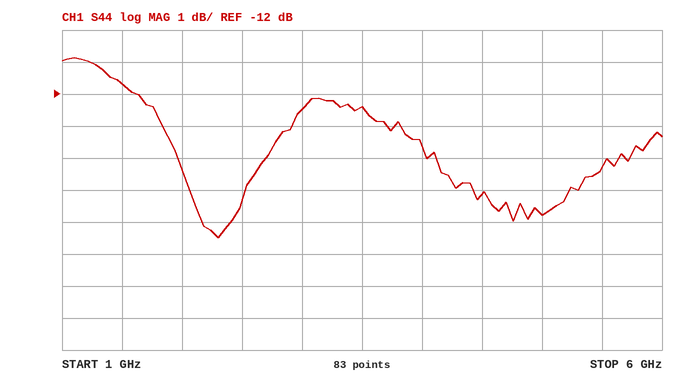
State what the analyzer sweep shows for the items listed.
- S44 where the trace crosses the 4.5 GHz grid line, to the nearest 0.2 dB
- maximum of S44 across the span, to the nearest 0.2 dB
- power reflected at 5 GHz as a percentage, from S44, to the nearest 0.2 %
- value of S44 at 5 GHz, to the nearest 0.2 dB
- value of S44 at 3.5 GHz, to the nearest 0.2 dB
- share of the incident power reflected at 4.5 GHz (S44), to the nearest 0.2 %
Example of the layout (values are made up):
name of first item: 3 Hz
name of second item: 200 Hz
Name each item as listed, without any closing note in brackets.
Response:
S44 where the trace crosses the 4.5 GHz grid line, to the nearest 0.2 dB: -15.2 dB
maximum of S44 across the span, to the nearest 0.2 dB: -10.8 dB
power reflected at 5 GHz as a percentage, from S44, to the nearest 0.2 %: 2.6 %
value of S44 at 5 GHz, to the nearest 0.2 dB: -15.8 dB
value of S44 at 3.5 GHz, to the nearest 0.2 dB: -12.4 dB
share of the incident power reflected at 4.5 GHz (S44), to the nearest 0.2 %: 3.0 %
